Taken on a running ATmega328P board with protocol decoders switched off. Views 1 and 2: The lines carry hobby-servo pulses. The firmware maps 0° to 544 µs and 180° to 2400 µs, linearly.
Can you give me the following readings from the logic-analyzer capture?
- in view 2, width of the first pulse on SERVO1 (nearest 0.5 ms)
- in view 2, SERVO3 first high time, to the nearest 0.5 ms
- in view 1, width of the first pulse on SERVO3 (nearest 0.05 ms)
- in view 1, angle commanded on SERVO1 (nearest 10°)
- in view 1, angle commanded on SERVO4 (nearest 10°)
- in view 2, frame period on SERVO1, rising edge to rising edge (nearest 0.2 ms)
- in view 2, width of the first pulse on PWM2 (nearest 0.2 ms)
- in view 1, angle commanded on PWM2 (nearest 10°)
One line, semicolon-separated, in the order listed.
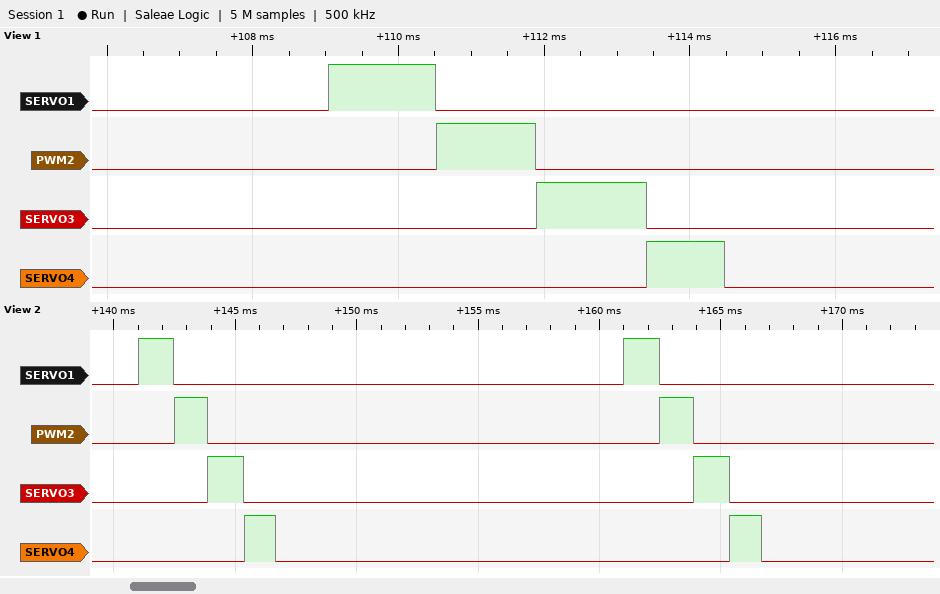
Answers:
1.5 ms; 1.5 ms; 1.50 ms; 90°; 50°; 20.0 ms; 1.4 ms; 80°
